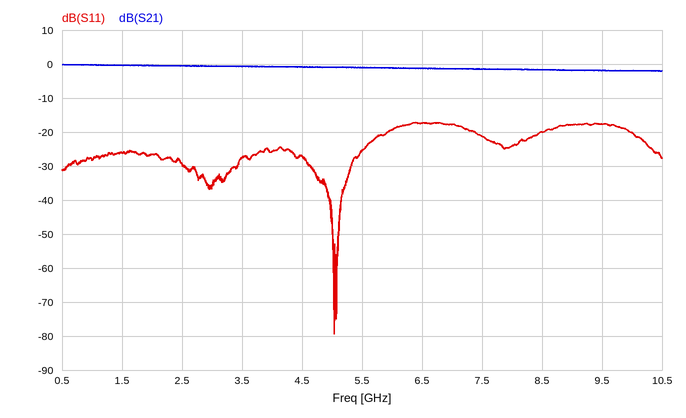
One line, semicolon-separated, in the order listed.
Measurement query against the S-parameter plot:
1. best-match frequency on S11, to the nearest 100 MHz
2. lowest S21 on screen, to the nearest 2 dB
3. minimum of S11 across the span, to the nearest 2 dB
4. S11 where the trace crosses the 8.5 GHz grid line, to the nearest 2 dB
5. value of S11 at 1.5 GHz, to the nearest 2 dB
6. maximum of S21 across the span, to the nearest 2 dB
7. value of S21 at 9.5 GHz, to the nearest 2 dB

5.0 GHz; -2 dB; -80 dB; -20 dB; -26 dB; 0 dB; -2 dB
